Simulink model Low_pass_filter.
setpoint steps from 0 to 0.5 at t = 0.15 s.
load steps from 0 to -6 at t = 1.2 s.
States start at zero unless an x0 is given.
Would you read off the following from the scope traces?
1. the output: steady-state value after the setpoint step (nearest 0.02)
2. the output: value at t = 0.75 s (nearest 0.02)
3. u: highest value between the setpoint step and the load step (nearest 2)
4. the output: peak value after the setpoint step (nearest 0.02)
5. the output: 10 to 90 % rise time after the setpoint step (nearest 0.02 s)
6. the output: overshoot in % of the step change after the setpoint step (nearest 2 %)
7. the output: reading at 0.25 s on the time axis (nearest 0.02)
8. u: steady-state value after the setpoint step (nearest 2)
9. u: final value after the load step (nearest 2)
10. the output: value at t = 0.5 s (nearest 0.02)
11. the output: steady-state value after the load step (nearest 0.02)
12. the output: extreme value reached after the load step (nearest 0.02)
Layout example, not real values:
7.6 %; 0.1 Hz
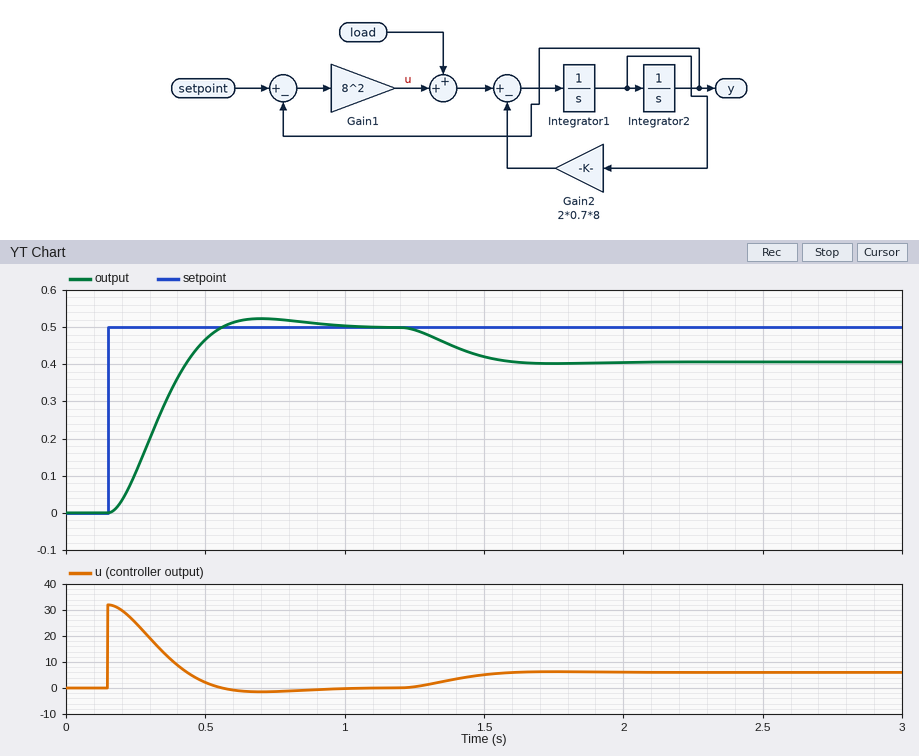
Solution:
0.50; 0.52; 32; 0.52; 0.26 s; 4 %; 0.10; 0; 6; 0.46; 0.40; 0.40
